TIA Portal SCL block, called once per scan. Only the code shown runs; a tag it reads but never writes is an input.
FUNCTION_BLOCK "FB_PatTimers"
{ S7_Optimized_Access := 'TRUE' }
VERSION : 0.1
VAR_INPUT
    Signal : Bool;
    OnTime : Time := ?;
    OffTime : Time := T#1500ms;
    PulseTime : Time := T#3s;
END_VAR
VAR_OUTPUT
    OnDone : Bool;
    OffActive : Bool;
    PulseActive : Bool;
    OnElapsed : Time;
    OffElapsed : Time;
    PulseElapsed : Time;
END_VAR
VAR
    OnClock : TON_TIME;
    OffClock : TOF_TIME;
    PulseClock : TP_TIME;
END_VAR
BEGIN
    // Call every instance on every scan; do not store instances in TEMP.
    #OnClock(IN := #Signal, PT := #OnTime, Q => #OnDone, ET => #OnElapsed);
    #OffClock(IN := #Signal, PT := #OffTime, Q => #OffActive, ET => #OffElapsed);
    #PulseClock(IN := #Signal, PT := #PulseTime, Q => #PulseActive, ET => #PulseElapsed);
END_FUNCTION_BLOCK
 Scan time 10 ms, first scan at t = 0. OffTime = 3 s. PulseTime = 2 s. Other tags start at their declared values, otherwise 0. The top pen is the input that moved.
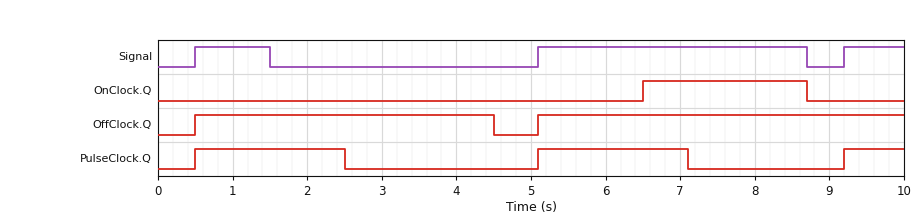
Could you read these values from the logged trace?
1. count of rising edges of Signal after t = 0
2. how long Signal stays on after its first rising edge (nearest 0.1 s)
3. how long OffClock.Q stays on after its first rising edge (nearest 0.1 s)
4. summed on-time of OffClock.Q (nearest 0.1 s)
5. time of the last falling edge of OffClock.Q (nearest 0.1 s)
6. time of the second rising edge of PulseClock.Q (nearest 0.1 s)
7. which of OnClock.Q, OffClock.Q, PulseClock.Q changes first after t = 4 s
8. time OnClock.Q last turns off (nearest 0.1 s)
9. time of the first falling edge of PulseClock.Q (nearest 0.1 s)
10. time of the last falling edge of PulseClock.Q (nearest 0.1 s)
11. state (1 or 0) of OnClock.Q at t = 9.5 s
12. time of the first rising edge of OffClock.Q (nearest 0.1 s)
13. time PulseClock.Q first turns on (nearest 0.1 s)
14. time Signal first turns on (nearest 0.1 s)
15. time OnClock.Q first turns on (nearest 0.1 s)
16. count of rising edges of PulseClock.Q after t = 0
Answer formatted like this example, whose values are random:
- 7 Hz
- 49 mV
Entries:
- 3
- 1.0 s
- 4.0 s
- 8.9 s
- 4.5 s
- 5.1 s
- OffClock.Q
- 8.7 s
- 2.5 s
- 7.1 s
- 0
- 0.5 s
- 0.5 s
- 0.5 s
- 6.5 s
- 3
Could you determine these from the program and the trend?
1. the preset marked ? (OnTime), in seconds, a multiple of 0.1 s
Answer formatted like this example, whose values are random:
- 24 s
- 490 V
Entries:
- 1.4 s
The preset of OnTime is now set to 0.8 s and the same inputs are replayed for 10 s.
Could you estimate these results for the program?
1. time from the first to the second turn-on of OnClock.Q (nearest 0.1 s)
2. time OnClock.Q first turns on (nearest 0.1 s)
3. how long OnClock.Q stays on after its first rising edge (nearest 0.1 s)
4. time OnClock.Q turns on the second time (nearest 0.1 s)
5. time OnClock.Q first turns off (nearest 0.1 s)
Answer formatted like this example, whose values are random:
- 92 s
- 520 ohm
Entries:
- 4.6 s
- 1.3 s
- 0.2 s
- 5.9 s
- 1.5 s
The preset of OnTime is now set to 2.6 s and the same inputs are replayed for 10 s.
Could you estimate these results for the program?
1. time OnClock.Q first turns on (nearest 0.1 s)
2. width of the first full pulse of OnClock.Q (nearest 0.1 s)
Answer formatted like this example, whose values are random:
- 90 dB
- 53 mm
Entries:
- 7.7 s
- 1.0 s
